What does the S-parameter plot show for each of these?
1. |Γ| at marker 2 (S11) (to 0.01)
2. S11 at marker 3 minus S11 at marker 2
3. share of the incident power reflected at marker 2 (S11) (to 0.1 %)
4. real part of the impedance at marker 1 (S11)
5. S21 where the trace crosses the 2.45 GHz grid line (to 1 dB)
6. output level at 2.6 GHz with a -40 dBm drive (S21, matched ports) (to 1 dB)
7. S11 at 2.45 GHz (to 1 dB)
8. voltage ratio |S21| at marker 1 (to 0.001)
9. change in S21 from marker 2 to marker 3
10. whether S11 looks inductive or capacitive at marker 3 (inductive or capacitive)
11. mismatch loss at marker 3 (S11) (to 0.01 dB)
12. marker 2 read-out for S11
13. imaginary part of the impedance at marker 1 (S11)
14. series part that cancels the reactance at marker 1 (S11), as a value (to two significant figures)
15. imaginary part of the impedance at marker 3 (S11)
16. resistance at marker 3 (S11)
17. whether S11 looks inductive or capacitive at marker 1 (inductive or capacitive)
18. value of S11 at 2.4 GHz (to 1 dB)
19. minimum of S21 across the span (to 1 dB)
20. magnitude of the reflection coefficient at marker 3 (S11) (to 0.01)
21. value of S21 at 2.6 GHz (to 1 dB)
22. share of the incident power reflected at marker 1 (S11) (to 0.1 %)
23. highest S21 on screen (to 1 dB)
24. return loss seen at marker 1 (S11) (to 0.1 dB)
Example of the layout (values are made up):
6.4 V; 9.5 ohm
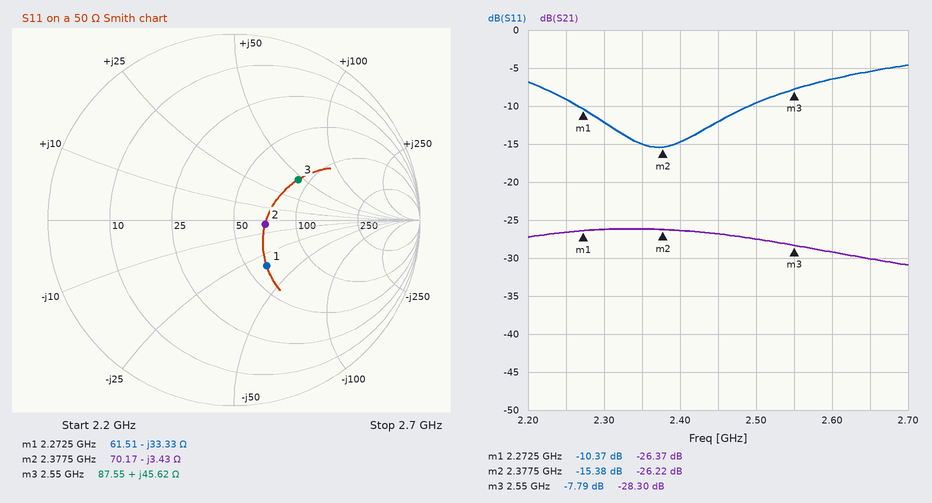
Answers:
0.17; 7.59 dB; 2.9 %; 61.51 Ω; -27 dB; -69 dBm; -12 dB; 0.048; -2.08 dB; inductive; 0.79 dB; -15.38 dB; -33.33 Ω; 2.3 nH; +45.62 Ω; 87.55 Ω; capacitive; -15 dB; -31 dB; 0.41; -29 dB; 9.2 %; -26 dB; 10.4 dB
